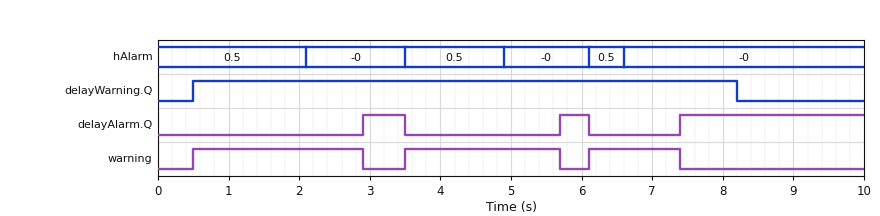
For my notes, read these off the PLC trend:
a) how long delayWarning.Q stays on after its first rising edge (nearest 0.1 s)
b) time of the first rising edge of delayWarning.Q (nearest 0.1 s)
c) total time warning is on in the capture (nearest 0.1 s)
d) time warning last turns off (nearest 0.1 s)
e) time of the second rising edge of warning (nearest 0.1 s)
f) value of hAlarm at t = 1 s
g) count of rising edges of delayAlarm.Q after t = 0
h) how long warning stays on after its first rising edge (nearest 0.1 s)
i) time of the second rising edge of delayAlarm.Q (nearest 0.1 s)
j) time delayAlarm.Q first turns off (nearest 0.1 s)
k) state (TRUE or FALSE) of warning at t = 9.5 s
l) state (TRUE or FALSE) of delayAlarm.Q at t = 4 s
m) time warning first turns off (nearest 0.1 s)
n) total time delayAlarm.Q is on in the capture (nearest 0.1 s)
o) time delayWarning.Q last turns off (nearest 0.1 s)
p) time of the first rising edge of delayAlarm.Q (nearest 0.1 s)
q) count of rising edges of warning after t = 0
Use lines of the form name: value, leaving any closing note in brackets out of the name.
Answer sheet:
how long delayWarning.Q stays on after its first rising edge: 7.7 s
time of the first rising edge of delayWarning.Q: 0.5 s
total time warning is on in the capture: 5.9 s
time warning last turns off: 7.4 s
time of the second rising edge of warning: 3.5 s
value of hAlarm at t = 1 s: 0.5
count of rising edges of delayAlarm.Q after t = 0: 3
how long warning stays on after its first rising edge: 2.4 s
time of the second rising edge of delayAlarm.Q: 5.7 s
time delayAlarm.Q first turns off: 3.5 s
state (TRUE or FALSE) of warning at t = 9.5 s: FALSE
state (TRUE or FALSE) of delayAlarm.Q at t = 4 s: FALSE
time warning first turns off: 2.9 s
total time delayAlarm.Q is on in the capture: 3.6 s
time delayWarning.Q last turns off: 8.2 s
time of the first rising edge of delayAlarm.Q: 2.9 s
count of rising edges of warning after t = 0: 3
